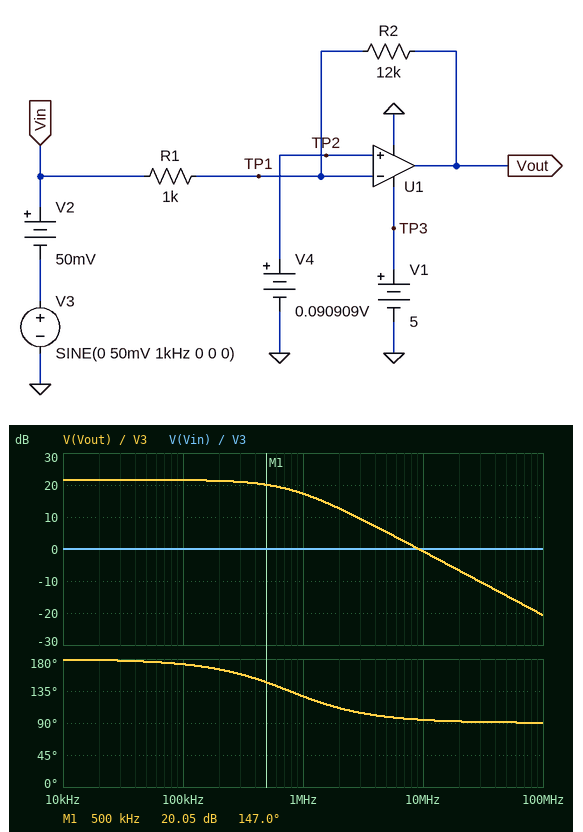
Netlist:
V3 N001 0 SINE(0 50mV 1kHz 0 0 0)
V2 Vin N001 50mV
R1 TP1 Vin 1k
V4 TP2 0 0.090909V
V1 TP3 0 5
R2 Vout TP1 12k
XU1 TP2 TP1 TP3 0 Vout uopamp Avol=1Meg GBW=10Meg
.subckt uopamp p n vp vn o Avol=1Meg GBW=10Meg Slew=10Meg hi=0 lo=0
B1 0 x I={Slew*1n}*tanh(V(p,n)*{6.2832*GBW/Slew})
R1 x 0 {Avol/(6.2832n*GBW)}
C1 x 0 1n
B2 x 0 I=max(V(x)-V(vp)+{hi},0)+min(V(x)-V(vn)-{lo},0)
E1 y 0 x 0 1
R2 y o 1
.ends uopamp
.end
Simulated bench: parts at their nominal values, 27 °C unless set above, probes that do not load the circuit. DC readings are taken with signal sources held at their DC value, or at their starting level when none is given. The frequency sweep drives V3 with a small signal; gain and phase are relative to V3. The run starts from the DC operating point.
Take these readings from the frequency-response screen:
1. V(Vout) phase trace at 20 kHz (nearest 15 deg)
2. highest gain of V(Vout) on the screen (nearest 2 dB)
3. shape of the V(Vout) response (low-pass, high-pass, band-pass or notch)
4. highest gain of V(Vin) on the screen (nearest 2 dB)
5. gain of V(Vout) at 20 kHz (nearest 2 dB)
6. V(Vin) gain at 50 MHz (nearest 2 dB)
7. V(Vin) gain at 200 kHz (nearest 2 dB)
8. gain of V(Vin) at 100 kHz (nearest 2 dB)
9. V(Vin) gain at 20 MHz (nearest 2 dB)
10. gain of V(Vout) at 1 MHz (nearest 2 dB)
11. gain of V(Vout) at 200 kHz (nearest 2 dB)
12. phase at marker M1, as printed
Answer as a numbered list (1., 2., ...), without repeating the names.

1. 180 deg
2. 22 dB
3. low-pass
4. 0 dB
5. 22 dB
6. 0 dB
7. 0 dB
8. 0 dB
9. 0 dB
10. 18 dB
11. 22 dB
12. 147.0 deg
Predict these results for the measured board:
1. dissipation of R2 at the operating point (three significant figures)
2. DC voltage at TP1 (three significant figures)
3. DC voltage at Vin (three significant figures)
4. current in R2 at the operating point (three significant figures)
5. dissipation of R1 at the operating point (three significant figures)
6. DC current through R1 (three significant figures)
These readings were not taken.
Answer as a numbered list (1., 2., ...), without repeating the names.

1. 20.1 µW
2. 90.9 mV
3. 50.0 mV
4. 40.9 µA
5. 1.67 µW
6. 40.9 µA
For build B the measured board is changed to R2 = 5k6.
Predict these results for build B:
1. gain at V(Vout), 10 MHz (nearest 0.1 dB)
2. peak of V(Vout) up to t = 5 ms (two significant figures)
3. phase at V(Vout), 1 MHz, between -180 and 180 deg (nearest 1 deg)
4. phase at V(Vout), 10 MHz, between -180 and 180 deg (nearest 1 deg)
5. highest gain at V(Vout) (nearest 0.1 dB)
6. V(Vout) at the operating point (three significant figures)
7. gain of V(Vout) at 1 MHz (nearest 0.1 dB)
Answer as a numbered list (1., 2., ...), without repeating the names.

1. -1.5 dB
2. 600 mV
3. 147 deg
4. 99 deg
5. 15.0 dB
6. 320 mV
7. 13.4 dB
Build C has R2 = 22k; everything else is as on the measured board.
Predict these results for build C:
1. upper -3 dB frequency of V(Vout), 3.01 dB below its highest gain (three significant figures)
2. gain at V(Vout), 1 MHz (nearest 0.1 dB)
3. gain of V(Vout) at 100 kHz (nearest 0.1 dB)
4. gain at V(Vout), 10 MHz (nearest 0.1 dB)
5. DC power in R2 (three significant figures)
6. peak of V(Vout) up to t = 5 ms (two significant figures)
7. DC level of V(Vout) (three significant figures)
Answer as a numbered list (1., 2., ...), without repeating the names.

1. 435 kHz
2. 18.9 dB
3. 26.6 dB
4. -0.4 dB
5. 36.8 µW
6. 2.1 V
7. 991 mV
